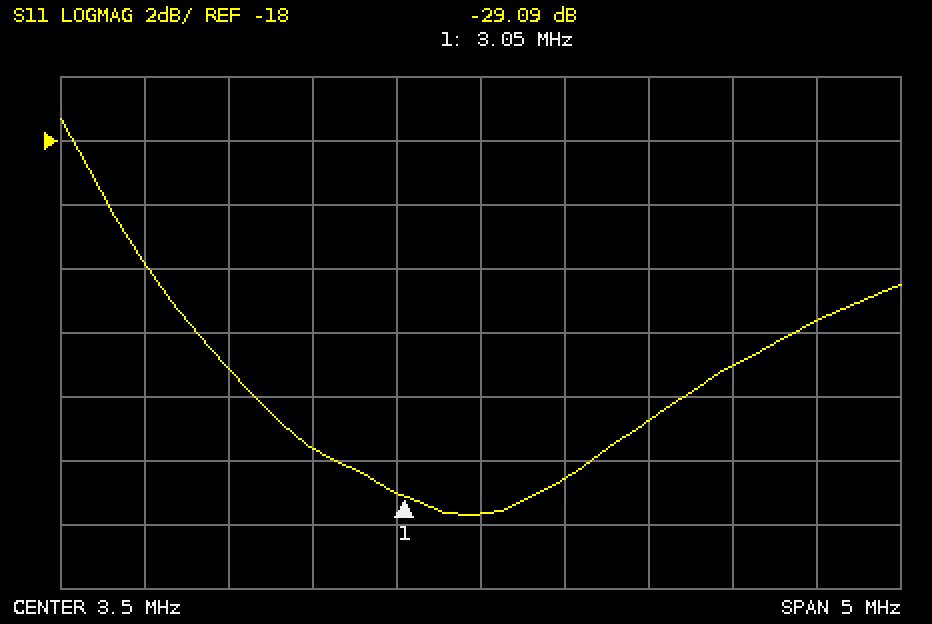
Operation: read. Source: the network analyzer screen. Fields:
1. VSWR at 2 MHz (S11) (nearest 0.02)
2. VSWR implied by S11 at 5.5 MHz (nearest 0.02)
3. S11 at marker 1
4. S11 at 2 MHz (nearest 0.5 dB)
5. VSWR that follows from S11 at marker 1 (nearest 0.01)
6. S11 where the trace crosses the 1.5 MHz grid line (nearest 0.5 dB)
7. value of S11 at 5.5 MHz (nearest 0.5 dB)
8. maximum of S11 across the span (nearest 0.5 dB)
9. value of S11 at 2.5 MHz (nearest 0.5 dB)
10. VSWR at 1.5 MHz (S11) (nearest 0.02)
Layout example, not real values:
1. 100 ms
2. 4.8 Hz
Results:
1. 1.12
2. 1.14
3. -29.09 dB
4. -25.0 dB
5. 1.07
6. -22.0 dB
7. -23.5 dB
8. -17.5 dB
9. -27.5 dB
10. 1.18
